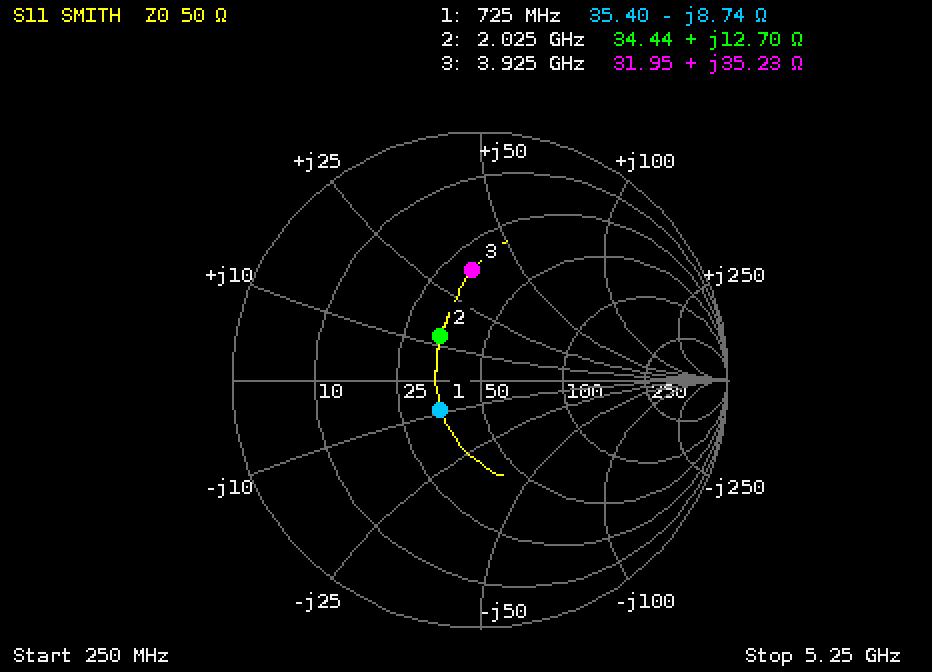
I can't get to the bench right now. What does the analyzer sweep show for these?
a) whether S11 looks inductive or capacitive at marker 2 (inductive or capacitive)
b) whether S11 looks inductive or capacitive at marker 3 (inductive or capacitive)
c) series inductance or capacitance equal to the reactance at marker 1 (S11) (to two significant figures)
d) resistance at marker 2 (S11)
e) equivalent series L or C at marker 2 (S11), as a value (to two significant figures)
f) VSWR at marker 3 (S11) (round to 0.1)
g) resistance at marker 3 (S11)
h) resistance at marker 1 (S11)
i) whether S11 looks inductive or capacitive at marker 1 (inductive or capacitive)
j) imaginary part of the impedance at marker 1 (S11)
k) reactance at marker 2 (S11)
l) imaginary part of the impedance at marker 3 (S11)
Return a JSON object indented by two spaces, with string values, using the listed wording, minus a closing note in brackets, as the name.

{
  "whether S11 looks inductive or capacitive at marker 2": "inductive",
  "whether S11 looks inductive or capacitive at marker 3": "inductive",
  "series inductance or capacitance equal to the reactance at marker 1 (S11)": "25 pF",
  "resistance at marker 2": "34.44 Ω",
  "equivalent series L or C at marker 2 (S11), as a value": "1.00 nH",
  "VSWR at marker 3 (S11)": "2.6",
  "resistance at marker 3": "31.95 Ω",
  "resistance at marker 1": "35.40 Ω",
  "whether S11 looks inductive or capacitive at marker 1": "capacitive",
  "imaginary part of the impedance at marker 1": "-8.74 Ω",
  "reactance at marker 2": "+12.70 Ω",
  "imaginary part of the impedance at marker 3": "+35.23 Ω"
}
